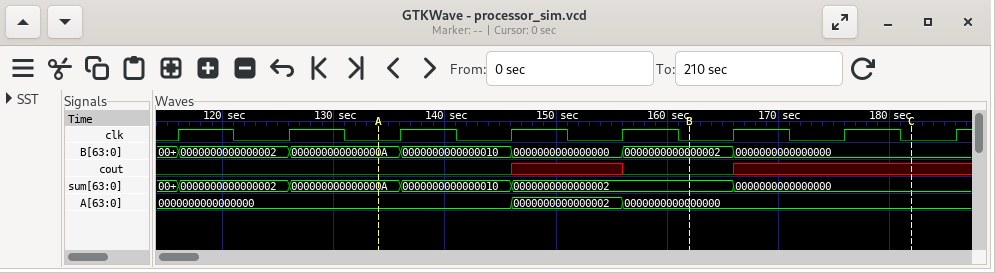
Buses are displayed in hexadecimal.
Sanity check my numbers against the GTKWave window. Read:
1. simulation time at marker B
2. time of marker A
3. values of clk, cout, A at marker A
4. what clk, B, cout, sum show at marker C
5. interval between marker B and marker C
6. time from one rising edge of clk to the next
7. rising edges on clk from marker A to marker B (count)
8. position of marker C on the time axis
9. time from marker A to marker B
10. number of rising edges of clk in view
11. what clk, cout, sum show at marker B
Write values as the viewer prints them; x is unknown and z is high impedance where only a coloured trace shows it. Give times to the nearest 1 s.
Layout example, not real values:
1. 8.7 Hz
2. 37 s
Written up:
1. 162 s
2. 134 s
3. clk=0, cout=0, A=0000000000000000
4. clk=0, B=0000000000000000, cout=x, sum=0000000000000000
5. 20 s
6. 10 s
7. 3
8. 182 s
9. 28 s
10. 8
11. clk=0, cout=0, sum=0000000000000002
